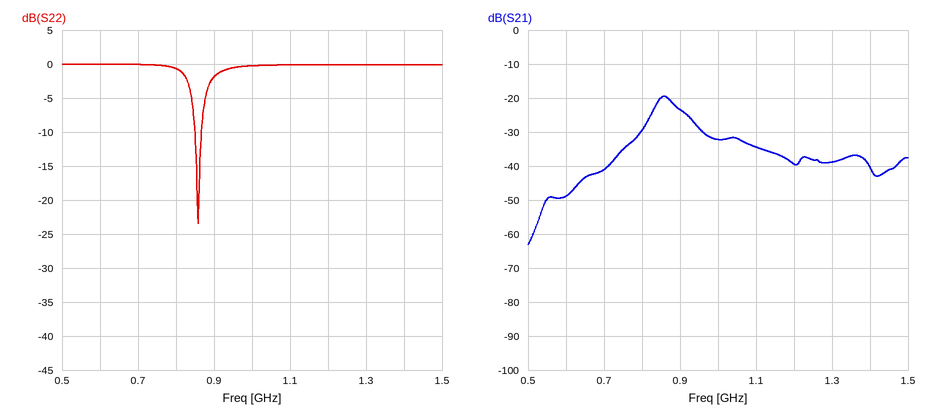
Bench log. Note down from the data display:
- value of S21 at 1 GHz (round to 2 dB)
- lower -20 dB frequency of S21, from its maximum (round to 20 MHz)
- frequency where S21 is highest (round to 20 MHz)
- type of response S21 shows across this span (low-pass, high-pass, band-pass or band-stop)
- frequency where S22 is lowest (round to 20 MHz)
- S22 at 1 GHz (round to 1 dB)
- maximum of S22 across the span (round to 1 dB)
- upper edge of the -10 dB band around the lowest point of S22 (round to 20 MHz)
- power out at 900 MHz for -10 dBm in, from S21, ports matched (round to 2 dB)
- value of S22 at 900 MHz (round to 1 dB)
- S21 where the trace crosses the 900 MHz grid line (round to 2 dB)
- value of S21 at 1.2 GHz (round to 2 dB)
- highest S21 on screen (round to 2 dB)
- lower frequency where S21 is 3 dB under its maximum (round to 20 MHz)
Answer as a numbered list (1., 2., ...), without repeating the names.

1. -32 dB
2. 720 MHz
3. 860 MHz
4. band-pass
5. 860 MHz
6. 0 dB
7. 0 dB
8. 860 MHz
9. -34 dBm
10. -2 dB
11. -24 dB
12. -40 dB
13. -20 dB
14. 840 MHz
